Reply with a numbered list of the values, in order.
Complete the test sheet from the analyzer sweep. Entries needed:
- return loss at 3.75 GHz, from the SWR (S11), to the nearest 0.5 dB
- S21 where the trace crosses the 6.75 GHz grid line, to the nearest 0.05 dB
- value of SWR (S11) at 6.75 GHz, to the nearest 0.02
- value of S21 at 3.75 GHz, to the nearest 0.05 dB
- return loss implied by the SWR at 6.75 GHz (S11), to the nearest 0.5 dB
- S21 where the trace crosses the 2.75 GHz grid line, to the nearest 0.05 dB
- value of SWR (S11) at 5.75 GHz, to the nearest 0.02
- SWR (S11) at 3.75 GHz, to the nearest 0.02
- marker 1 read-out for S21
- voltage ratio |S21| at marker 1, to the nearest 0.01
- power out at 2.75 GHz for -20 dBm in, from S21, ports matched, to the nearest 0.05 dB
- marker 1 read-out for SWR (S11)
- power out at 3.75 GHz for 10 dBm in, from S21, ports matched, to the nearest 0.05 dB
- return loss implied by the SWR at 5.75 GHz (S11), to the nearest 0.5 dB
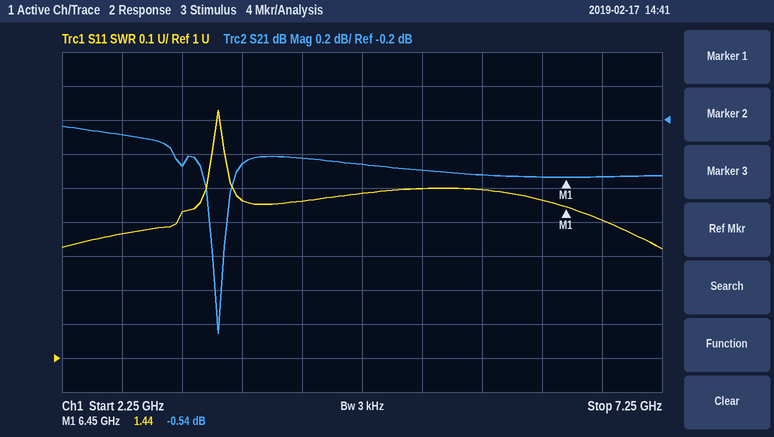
1. 14.5 dB
2. -0.55 dB
3. 1.40
4. -0.45 dB
5. 15.5 dB
6. -0.30 dB
7. 1.50
8. 1.46
9. -0.54 dB
10. 0.94
11. -20.30 dBm
12. 1.44
13. 9.55 dBm
14. 14.0 dB
